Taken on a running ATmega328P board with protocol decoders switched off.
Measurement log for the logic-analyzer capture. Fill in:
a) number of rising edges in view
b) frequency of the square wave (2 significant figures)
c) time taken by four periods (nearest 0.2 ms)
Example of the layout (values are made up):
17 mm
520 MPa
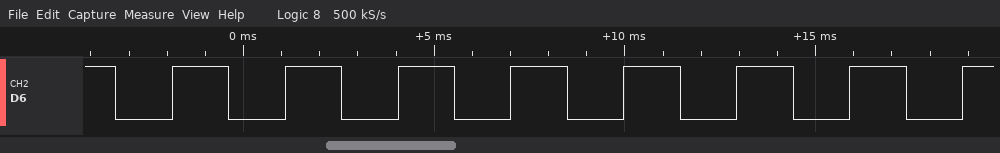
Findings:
8
340 Hz
11.8 ms
